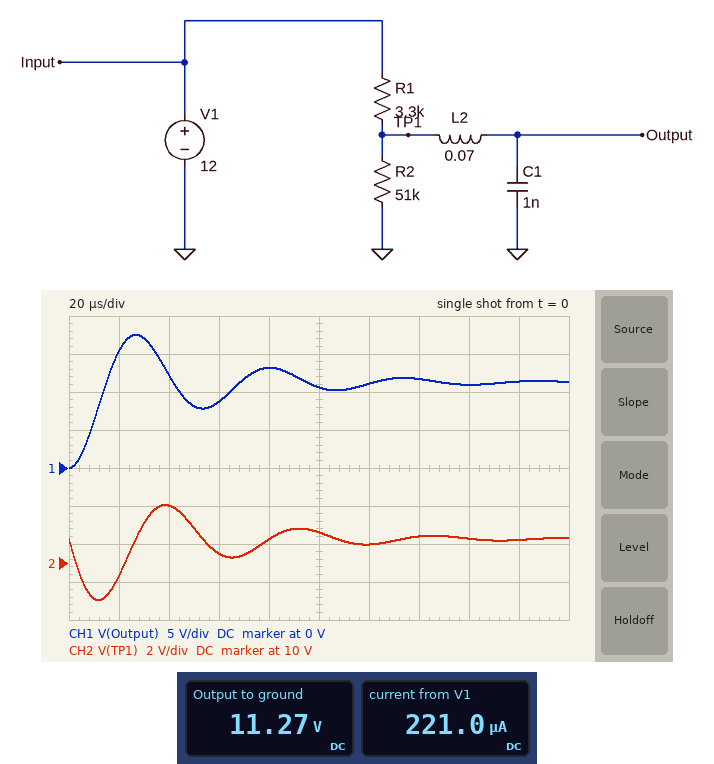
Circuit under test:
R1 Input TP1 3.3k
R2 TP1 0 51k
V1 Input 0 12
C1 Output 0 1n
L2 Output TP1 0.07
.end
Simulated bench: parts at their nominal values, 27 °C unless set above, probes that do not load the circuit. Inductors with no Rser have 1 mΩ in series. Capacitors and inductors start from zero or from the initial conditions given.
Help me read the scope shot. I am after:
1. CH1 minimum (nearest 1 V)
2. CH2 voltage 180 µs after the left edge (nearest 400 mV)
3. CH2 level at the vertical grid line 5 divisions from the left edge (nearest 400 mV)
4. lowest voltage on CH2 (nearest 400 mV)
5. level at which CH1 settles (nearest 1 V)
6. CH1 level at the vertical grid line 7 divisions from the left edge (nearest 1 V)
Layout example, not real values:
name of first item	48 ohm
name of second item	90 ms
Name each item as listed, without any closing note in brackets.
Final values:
CH1 minimum	0 V
CH2 voltage 180 µs after the left edge	11.2 V
CH2 level at the vertical grid line 5 divisions from the left edge	11.6 V
lowest voltage on CH2	8.0 V
level at which CH1 settles	11 V
CH1 level at the vertical grid line 7 divisions from the left edge	12 V
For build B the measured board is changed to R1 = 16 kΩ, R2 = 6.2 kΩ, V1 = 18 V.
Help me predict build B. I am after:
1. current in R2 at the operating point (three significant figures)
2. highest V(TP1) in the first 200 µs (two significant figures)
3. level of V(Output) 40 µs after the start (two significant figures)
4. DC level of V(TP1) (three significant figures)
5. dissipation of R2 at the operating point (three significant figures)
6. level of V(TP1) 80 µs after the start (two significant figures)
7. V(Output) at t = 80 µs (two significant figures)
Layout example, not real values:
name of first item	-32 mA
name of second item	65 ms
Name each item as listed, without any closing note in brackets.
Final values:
current in R2 at the operating point	811 µA
highest V(TP1) in the first 200 µs	5.8 V
level of V(Output) 40 µs after the start	5.6 V
DC level of V(TP1)	5.03 V
dissipation of R2 at the operating point	4.08 mW
level of V(TP1) 80 µs after the start	5.0 V
V(Output) at t = 80 µs	5.4 V
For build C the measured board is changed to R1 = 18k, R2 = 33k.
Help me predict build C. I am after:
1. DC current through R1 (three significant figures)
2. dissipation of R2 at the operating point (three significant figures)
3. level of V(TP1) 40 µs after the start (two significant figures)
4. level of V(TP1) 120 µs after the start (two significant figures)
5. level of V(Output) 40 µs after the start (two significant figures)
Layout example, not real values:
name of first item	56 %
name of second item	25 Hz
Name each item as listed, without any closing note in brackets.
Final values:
DC current through R1	235 µA
dissipation of R2 at the operating point	1.83 mW
level of V(TP1) 40 µs after the start	7.9 V
level of V(TP1) 120 µs after the start	7.8 V
level of V(Output) 40 µs after the start	8.1 V
